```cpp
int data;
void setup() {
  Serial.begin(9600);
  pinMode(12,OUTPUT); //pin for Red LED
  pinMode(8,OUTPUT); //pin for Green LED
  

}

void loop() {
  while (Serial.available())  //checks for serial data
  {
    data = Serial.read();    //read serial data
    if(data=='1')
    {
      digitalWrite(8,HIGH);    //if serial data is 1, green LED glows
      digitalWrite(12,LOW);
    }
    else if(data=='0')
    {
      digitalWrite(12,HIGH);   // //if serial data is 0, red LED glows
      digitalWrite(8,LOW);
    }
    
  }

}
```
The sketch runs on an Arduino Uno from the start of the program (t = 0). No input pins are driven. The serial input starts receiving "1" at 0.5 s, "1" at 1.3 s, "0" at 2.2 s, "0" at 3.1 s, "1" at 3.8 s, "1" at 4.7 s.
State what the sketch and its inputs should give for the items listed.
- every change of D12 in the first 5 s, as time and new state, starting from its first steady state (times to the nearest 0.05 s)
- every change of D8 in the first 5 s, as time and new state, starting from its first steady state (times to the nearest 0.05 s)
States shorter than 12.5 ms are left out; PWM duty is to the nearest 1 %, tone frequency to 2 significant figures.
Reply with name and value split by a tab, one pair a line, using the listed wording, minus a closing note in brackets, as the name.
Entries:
every change of D12 in the first 5 s, as time and new state, starting from its first steady state	0 s low; 2.2 s high; 3.8 s low
every change of D8 in the first 5 s, as time and new state, starting from its first steady state	0 s low; 0.5 s high; 2.2 s low; 3.8 s high
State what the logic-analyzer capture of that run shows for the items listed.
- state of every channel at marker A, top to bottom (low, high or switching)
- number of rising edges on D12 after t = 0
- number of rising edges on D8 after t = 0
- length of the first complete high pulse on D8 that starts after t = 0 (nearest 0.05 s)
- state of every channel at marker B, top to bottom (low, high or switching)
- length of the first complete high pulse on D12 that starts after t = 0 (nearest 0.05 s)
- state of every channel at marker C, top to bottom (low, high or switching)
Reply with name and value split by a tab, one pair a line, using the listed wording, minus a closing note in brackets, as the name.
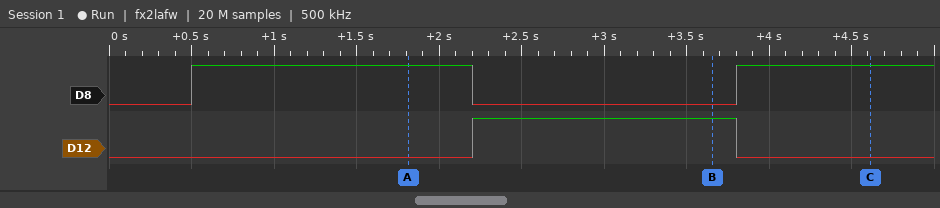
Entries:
state of every channel at marker A, top to bottom	D8 high, D12 low
number of rising edges on D12 after t = 0	1
number of rising edges on D8 after t = 0	2
length of the first complete high pulse on D8 that starts after t = 0	1.70 s
state of every channel at marker B, top to bottom	D8 low, D12 high
length of the first complete high pulse on D12 that starts after t = 0	1.60 s
state of every channel at marker C, top to bottom	D8 high, D12 low
